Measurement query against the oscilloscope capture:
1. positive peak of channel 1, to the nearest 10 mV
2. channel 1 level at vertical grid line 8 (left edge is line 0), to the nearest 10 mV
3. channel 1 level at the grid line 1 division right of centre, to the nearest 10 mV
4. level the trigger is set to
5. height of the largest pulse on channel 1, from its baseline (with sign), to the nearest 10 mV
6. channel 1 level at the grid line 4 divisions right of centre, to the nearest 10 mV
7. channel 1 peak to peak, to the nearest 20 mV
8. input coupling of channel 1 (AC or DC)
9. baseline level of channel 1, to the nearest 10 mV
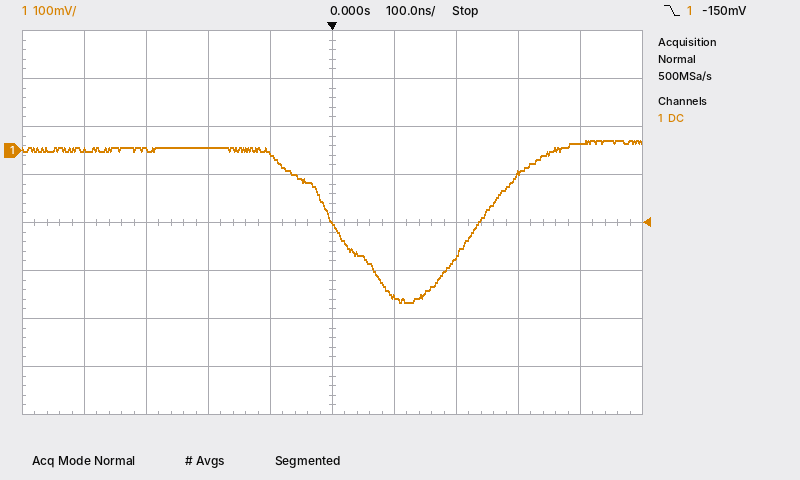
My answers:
20 mV
-50 mV
-300 mV
-150 mV
-320 mV
10 mV
340 mV
DC
0 mV
